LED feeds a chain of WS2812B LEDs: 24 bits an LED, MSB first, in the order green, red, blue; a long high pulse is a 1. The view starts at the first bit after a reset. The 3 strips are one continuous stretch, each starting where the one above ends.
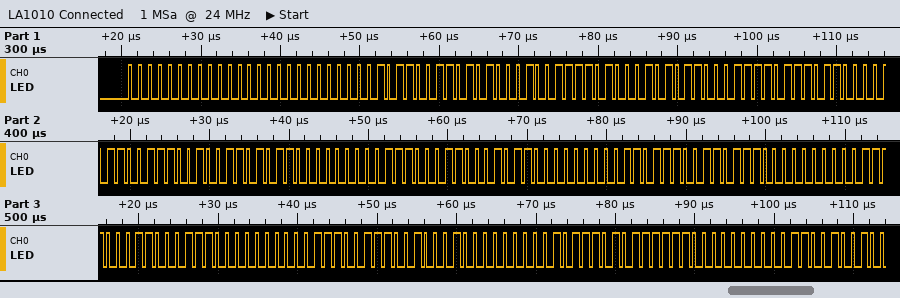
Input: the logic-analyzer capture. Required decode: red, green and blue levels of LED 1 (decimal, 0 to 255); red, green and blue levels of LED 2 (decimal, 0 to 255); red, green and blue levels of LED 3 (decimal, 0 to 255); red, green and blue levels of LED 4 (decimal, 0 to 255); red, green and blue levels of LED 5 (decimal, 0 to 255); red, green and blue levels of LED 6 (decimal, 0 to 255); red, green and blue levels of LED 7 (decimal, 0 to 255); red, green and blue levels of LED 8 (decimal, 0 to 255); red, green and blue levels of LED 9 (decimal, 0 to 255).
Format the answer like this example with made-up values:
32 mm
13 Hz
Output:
0, 0, 0
168, 89, 158
199, 138, 187
114, 6, 107
113, 0, 139
110, 0, 110
113, 0, 142
115, 0, 145
93, 0, 126
